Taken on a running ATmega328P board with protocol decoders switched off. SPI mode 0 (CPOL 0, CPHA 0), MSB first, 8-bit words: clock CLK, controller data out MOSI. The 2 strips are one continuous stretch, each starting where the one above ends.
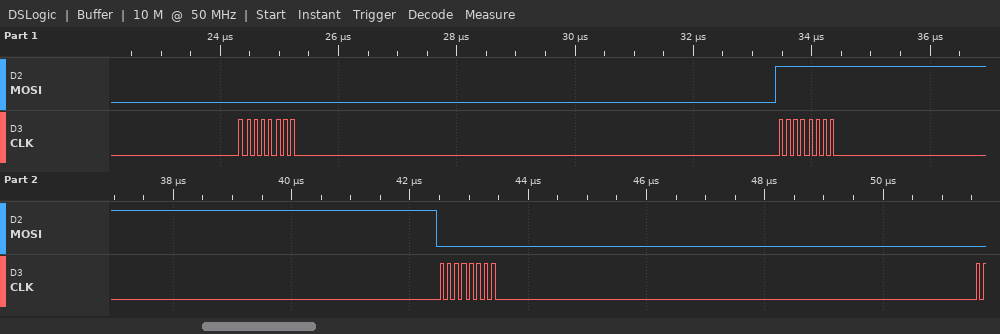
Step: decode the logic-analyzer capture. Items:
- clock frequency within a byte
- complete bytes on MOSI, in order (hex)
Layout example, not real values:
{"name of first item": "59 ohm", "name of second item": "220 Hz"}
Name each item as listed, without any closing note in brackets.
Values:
{"clock frequency within a byte": "8 MHz", "complete bytes on MOSI, in order": "0x00 0xFF 0x00"}
